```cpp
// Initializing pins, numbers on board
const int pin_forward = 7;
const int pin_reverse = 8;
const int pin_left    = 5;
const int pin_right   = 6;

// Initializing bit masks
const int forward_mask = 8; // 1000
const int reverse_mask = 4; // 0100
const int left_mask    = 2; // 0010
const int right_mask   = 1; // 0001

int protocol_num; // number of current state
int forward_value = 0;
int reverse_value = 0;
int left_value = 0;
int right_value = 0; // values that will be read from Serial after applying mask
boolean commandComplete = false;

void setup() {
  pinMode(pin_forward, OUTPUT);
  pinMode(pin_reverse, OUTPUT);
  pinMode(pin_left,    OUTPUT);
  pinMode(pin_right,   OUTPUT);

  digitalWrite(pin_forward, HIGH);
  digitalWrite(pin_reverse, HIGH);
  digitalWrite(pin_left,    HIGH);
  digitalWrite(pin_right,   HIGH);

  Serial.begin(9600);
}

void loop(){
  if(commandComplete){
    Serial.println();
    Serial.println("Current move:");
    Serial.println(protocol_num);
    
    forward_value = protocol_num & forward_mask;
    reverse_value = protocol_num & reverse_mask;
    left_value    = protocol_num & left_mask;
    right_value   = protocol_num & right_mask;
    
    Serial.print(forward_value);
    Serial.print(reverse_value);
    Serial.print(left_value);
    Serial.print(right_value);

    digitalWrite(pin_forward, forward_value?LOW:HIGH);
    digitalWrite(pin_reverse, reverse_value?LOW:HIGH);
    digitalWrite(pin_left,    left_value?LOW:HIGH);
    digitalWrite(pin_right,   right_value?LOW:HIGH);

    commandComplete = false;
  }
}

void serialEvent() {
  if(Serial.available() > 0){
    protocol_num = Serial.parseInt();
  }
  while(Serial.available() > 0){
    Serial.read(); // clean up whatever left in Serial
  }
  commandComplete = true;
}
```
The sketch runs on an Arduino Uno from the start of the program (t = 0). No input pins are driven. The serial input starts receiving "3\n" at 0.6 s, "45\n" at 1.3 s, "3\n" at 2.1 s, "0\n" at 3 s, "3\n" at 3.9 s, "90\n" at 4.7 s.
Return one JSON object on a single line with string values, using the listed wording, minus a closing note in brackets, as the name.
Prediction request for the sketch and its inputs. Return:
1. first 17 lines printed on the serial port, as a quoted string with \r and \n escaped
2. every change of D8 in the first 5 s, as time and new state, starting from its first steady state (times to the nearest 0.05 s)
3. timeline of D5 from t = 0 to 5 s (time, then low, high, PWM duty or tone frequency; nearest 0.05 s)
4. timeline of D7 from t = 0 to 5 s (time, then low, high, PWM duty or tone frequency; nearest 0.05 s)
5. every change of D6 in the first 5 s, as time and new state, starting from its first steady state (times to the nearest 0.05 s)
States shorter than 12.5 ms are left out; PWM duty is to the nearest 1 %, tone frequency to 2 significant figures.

{"first 17 lines printed on the serial port, as a quoted string with \\r and \\n escaped": "\"\\r\\nCurrent move:\\r\\n3\\r\\n0021\\r\\nCurrent move:\\r\\n45\\r\\n8401\\r\\nCurrent move:\\r\\n3\\r\\n0021\\r\\nCurrent move:\\r\\n0\\r\\n0000\\r\\nCurrent move:\\r\\n3\\r\\n0021\\r\\nCurrent move:\\r\\n\"", "every change of D8 in the first 5 s, as time and new state, starting from its first steady state": "0 s high; 1.3 s low; 2.1 s high", "timeline of D5 from t = 0 to 5 s": "0 s high; 0.6 s low; 1.3 s high; 2.1 s low; 3 s high; 3.9 s low", "timeline of D7 from t = 0 to 5 s": "0 s high; 1.3 s low; 2.1 s high; 4.7 s low", "every change of D6 in the first 5 s, as time and new state, starting from its first steady state": "0 s high; 0.6 s low; 3 s high; 3.9 s low; 4.7 s high"}
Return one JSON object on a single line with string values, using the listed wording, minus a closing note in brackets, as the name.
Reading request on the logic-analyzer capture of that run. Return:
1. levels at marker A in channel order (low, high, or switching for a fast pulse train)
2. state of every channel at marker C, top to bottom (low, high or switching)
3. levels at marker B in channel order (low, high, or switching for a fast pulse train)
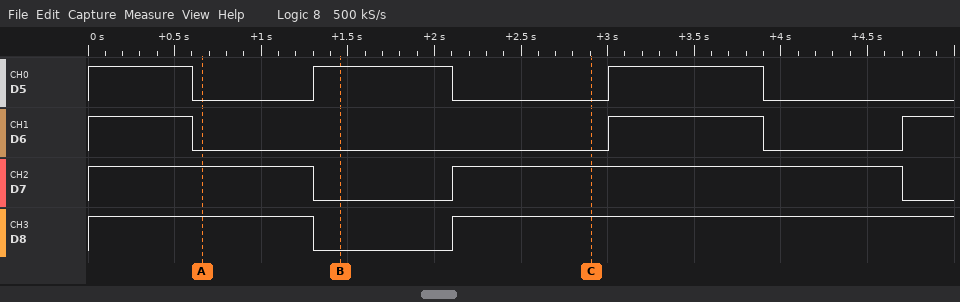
{"levels at marker A in channel order": "D5 low, D6 low, D7 high, D8 high", "state of every channel at marker C, top to bottom": "D5 low, D6 low, D7 high, D8 high", "levels at marker B in channel order": "D5 high, D6 low, D7 low, D8 low"}
